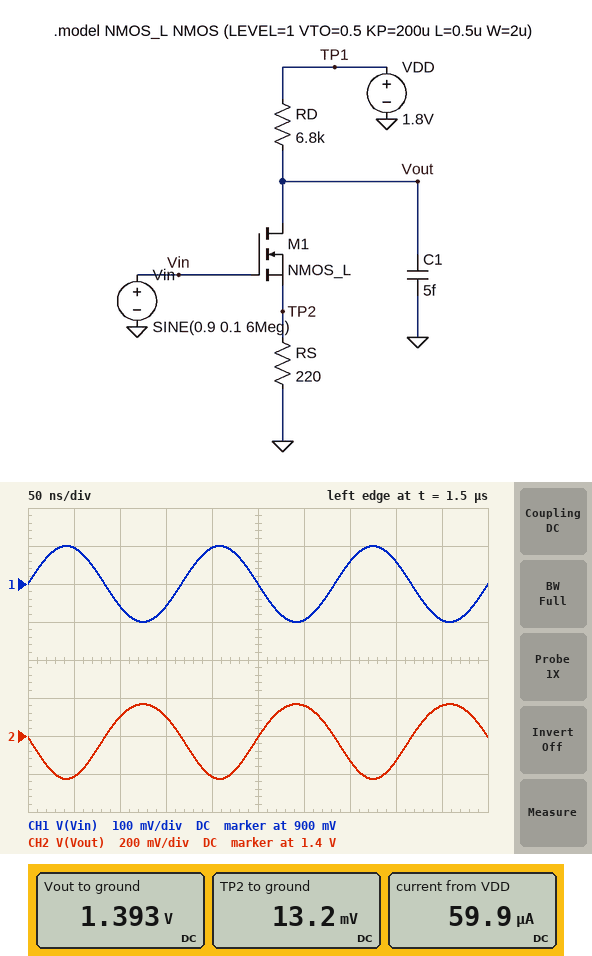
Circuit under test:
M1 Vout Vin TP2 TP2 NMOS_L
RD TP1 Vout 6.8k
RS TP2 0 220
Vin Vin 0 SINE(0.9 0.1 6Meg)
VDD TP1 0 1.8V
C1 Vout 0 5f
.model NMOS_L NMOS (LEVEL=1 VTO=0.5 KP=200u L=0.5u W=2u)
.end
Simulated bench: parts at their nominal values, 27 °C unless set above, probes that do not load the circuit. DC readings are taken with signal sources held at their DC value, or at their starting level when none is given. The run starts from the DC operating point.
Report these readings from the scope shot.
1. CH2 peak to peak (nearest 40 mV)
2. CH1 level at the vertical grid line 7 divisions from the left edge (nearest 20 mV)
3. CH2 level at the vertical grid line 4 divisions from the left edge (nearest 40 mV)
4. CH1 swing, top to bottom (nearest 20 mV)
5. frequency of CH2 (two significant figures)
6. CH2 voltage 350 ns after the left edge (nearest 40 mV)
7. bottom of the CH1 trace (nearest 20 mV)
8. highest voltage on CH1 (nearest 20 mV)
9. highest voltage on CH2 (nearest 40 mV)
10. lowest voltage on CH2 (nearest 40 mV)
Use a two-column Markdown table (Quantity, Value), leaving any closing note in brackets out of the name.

| Quantity | Value |
|---|---|
| CH2 peak to peak | 400 mV |
| CH1 level at the vertical grid line 7 divisions from the left edge | 960 mV |
| CH2 level at the vertical grid line 4 divisions from the left edge | 1.20 V |
| CH1 swing, top to bottom | 200 mV |
| frequency of CH2 | 6.0 MHz |
| CH2 voltage 350 ns after the left edge | 1.28 V |
| bottom of the CH1 trace | 800 mV |
| highest voltage on CH1 | 1.00 V |
| highest voltage on CH2 | 1.56 V |
| lowest voltage on CH2 | 1.16 V |
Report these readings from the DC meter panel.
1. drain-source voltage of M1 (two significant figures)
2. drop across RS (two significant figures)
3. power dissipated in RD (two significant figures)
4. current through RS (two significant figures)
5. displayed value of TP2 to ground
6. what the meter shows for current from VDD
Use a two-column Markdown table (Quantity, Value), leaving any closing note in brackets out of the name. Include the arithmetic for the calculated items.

| Quantity | Value |
|---|---|
| drain-source voltage of M1 | 1.393 V - 13.2 mV = 1.4 V |
| drop across RS | 13.2 mV = 13 mV |
| power dissipated in RD | (1.8 V - 1.393 V)^2 / 6.8 kΩ = 24 µW |
| current through RS | (13.2 mV) / 220 Ω = 60 µA |
| displayed value of TP2 to ground | 13.2 mV |
| what the meter shows for current from VDD | 59.9 µA |
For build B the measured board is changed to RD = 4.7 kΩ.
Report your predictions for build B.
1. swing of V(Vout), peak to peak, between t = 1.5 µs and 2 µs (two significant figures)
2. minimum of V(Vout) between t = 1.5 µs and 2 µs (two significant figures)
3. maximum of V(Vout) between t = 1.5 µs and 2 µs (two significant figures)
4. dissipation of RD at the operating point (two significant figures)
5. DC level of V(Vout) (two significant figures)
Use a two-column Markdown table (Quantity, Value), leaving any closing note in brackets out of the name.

| Quantity | Value |
|---|---|
| swing of V(Vout), peak to peak, between t = 1.5 µs and 2 µs | 270 mV |
| minimum of V(Vout) between t = 1.5 µs and 2 µs | 1.4 V |
| maximum of V(Vout) between t = 1.5 µs and 2 µs | 1.6 V |
| dissipation of RD at the operating point | 17 µW |
| DC level of V(Vout) | 1.5 V |
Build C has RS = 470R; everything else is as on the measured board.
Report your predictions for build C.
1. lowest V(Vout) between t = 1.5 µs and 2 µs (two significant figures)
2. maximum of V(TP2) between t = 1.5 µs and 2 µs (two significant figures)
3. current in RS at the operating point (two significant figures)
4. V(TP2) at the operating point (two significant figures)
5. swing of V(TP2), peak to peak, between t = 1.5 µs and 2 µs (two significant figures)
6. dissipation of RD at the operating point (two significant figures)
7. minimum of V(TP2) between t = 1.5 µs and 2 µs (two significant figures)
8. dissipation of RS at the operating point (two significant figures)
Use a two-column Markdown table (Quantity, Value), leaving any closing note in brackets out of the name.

| Quantity | Value |
|---|---|
| lowest V(Vout) between t = 1.5 µs and 2 µs | 1.2 V |
| maximum of V(TP2) between t = 1.5 µs and 2 µs | 40 mV |
| current in RS at the operating point | 56 µA |
| V(TP2) at the operating point | 26 mV |
| swing of V(TP2), peak to peak, between t = 1.5 µs and 2 µs | 25 mV |
| dissipation of RD at the operating point | 21 µW |
| minimum of V(TP2) between t = 1.5 µs and 2 µs | 15 mV |
| dissipation of RS at the operating point | 1.5 µW |
